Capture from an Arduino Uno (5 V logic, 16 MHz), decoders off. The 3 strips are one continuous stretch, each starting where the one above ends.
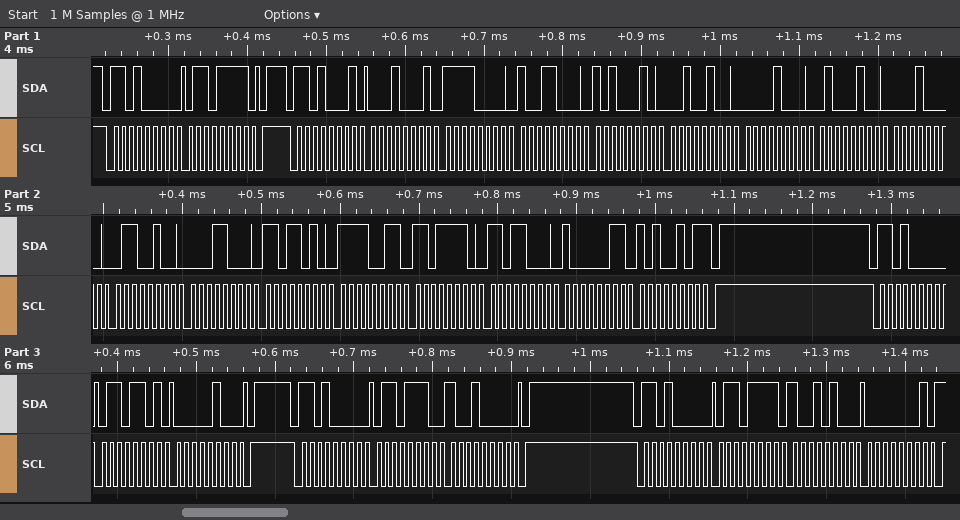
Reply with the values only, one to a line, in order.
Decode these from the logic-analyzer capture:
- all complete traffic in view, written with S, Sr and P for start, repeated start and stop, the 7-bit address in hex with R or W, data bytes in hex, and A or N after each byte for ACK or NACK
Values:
S 68W A 6F A P S 68R A 11 A F0 A 98 A A2 A 24 A 08 A 44 A 10 A 64 A 18 A DA A F3 A DE A D8 A 83 A A5 N P S 68W A 6D A 04 A P S 68W A 6E A 90 A P S 68W A 6F A 94 A 01 A
